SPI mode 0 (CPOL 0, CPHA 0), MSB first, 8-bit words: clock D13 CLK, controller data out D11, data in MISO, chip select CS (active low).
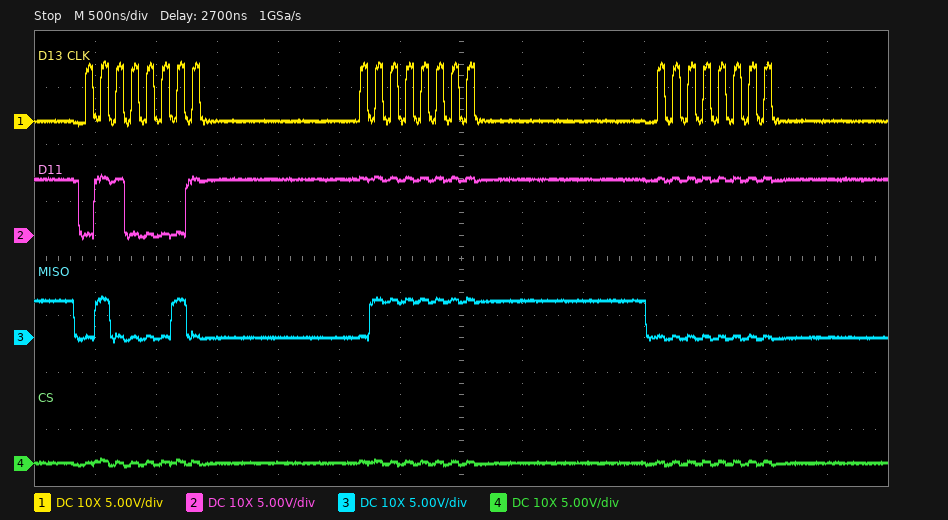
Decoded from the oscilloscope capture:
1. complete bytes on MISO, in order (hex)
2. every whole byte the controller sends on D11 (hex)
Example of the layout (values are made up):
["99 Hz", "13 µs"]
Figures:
["42 7F 00", "61 FF FF"]
